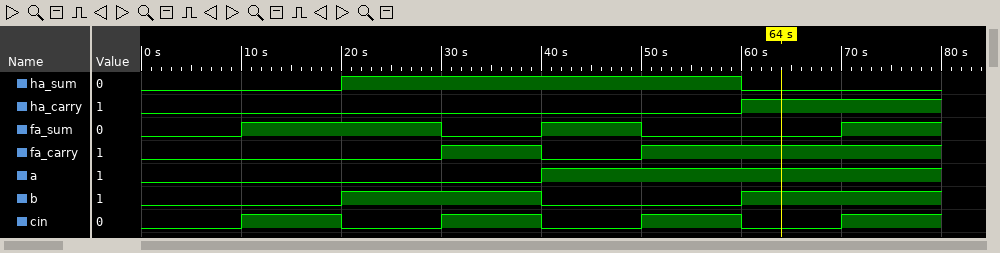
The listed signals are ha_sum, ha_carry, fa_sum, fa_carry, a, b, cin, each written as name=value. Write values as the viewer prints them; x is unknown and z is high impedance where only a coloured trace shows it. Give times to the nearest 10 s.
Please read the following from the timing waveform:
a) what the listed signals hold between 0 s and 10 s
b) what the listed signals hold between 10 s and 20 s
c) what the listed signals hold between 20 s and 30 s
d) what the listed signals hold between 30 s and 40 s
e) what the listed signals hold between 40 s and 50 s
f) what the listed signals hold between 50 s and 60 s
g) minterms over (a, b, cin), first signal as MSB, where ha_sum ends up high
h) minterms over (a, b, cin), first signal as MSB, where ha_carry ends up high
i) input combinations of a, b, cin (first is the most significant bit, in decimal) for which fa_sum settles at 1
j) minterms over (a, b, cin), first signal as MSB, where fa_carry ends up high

ha_sum=0, ha_carry=0, fa_sum=0, fa_carry=0, a=0, b=0, cin=0
ha_sum=0, ha_carry=0, fa_sum=1, fa_carry=0, a=0, b=0, cin=1
ha_sum=1, ha_carry=0, fa_sum=1, fa_carry=0, a=0, b=1, cin=0
ha_sum=1, ha_carry=0, fa_sum=0, fa_carry=1, a=0, b=1, cin=1
ha_sum=1, ha_carry=0, fa_sum=1, fa_carry=0, a=1, b=0, cin=0
ha_sum=1, ha_carry=0, fa_sum=0, fa_carry=1, a=1, b=0, cin=1
2, 3, 4, 5
6, 7
1, 2, 4, 7
3, 5, 6, 7
